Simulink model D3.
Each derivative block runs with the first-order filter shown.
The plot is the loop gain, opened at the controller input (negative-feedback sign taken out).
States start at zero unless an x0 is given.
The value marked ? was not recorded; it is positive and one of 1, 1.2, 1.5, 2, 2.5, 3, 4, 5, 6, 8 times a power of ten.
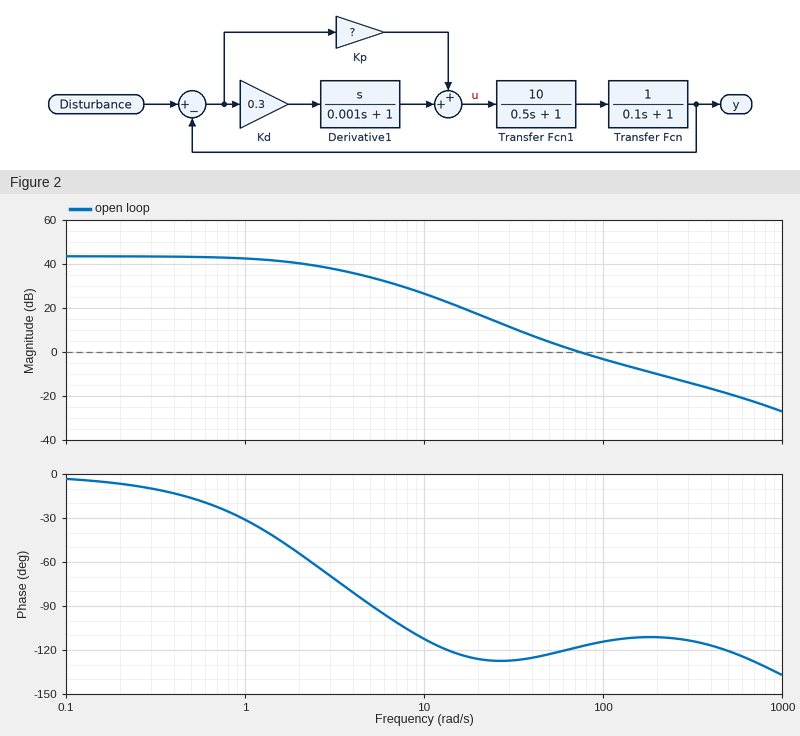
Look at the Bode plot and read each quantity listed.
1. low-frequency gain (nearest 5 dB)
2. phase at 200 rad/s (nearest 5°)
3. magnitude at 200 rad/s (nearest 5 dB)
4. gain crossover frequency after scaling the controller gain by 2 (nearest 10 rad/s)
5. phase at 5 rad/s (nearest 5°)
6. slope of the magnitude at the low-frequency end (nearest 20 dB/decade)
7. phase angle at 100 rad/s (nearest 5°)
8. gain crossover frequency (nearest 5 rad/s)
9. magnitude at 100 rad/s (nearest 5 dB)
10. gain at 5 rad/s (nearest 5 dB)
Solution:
45 dB
-110°
-10 dB
130 rad/s
-90°
0 dB/decade
-115°
75 rad/s
-5 dB
35 dB
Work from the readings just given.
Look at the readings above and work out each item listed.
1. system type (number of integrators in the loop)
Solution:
0
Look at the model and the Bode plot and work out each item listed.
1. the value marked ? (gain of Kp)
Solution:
15
